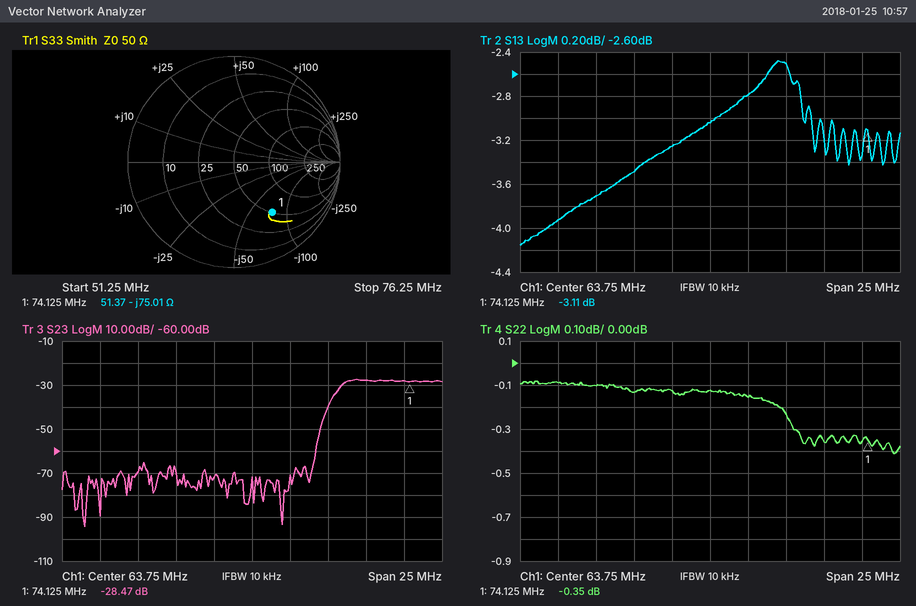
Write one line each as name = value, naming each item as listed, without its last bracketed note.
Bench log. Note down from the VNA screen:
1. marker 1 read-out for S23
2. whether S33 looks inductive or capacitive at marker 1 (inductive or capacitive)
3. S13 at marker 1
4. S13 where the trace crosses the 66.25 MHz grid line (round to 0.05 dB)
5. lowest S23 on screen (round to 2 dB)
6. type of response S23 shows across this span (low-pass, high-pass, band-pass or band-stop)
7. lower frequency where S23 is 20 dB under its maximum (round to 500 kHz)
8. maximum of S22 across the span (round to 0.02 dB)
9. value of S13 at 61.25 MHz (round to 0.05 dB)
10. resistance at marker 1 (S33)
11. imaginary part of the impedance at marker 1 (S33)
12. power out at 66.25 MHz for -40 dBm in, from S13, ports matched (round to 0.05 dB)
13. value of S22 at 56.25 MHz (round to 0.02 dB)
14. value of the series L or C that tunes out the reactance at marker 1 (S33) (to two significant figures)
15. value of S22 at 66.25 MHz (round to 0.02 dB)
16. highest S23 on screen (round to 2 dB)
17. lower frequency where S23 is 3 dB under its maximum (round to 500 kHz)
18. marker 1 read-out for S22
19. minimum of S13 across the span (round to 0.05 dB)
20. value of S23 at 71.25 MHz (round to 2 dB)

marker 1 read-out for S23 = -28.47 dB
whether S33 looks inductive or capacitive at marker 1 = capacitive
S13 at marker 1 = -3.11 dB
S13 where the trace crosses the 66.25 MHz grid line = -2.80 dB
lowest S23 on screen = -94 dB
type of response S23 shows across this span = high-pass
lower frequency where S23 is 20 dB under its maximum = 68.5 MHz
maximum of S22 across the span = -0.08 dB
value of S13 at 61.25 MHz = -3.25 dB
resistance at marker 1 = 51.37 Ω
imaginary part of the impedance at marker 1 = -75.01 Ω
power out at 66.25 MHz for -40 dBm in, from S13, ports matched = -42.80 dBm
value of S22 at 56.25 MHz = -0.10 dB
value of the series L or C that tunes out the reactance at marker 1 (S33) = 160 nH
value of S22 at 66.25 MHz = -0.16 dB
highest S23 on screen = -28 dB
lower frequency where S23 is 3 dB under its maximum = 69.5 MHz
marker 1 read-out for S22 = -0.35 dB
minimum of S13 across the span = -4.15 dB
value of S23 at 71.25 MHz = -28 dB
